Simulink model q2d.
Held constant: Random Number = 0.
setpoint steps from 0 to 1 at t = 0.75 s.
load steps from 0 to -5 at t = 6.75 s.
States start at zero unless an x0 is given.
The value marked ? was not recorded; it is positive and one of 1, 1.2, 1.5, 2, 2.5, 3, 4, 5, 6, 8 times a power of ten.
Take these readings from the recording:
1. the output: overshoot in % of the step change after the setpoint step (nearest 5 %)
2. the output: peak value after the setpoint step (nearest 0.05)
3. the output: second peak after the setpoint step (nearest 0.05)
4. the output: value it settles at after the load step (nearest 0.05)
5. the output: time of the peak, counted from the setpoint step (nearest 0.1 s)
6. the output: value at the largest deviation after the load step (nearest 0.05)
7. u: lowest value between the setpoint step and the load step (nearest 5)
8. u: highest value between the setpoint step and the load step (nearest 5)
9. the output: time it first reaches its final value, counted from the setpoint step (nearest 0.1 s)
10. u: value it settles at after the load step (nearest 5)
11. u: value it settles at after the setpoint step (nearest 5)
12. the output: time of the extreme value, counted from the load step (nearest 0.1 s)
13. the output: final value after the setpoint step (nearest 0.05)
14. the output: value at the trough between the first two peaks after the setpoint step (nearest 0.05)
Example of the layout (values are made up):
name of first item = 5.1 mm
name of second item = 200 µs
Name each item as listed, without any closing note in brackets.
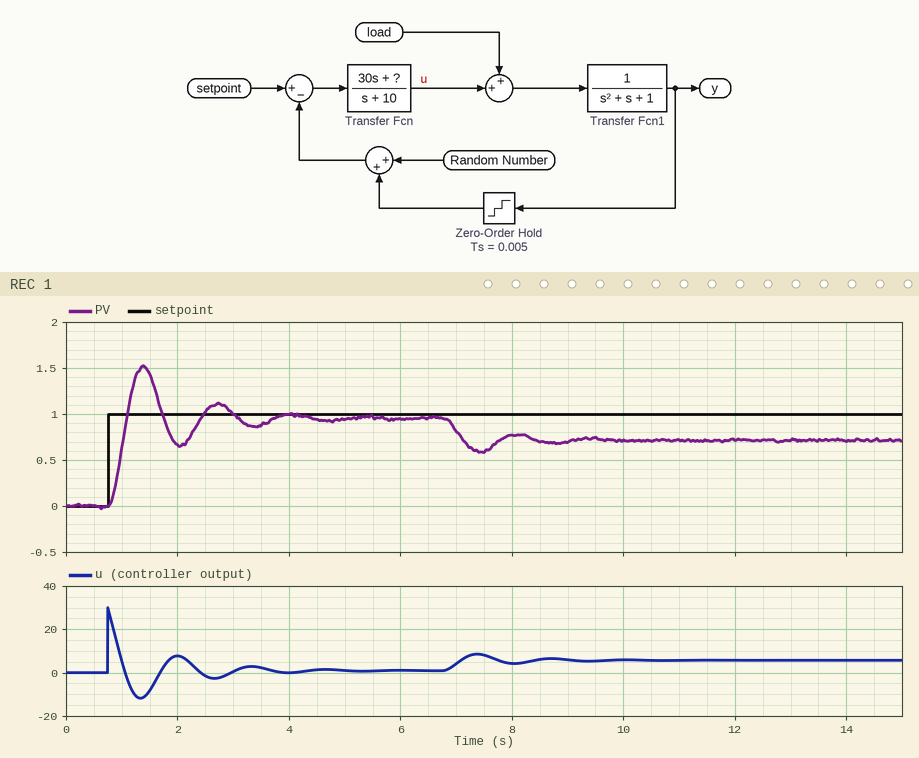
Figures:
the output: overshoot in % of the step change after the setpoint step = 60 %
the output: peak value after the setpoint step = 1.50
the output: second peak after the setpoint step = 1.10
the output: value it settles at after the load step = 0.70
the output: time of the peak, counted from the setpoint step = 0.6 s
the output: value at the largest deviation after the load step = 0.60
u: lowest value between the setpoint step and the load step = -10
u: highest value between the setpoint step and the load step = 30
the output: time it first reaches its final value, counted from the setpoint step = 0.3 s
u: value it settles at after the load step = 5
u: value it settles at after the setpoint step = 0
the output: time of the extreme value, counted from the load step = 0.7 s
the output: final value after the setpoint step = 0.95
the output: value at the trough between the first two peaks after the setpoint step = 0.65
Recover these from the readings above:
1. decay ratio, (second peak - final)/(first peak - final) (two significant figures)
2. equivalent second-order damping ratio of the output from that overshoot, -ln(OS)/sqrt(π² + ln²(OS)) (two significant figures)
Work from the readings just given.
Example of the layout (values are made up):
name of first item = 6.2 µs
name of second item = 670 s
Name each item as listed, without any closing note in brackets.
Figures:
decay ratio, (second peak - final)/(first peak - final) = 0.27
equivalent second-order damping ratio of the output from that overshoot, -ln(OS)/sqrt(π² + ln²(OS)) = 0.16
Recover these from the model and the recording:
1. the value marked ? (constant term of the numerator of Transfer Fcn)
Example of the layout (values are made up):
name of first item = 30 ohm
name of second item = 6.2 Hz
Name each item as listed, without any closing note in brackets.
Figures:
the value marked ? = 200
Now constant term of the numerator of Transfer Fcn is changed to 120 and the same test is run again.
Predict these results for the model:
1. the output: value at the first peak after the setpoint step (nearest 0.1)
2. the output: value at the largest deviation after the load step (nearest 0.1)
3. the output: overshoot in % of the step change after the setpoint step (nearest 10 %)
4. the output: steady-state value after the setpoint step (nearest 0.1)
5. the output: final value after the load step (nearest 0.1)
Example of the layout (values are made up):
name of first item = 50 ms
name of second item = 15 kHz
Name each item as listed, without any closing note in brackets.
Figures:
the output: value at the first peak after the setpoint step = 1.3
the output: value at the largest deviation after the load step = 0.4
the output: overshoot in % of the step change after the setpoint step = 40 %
the output: steady-state value after the setpoint step = 0.9
the output: final value after the load step = 0.5
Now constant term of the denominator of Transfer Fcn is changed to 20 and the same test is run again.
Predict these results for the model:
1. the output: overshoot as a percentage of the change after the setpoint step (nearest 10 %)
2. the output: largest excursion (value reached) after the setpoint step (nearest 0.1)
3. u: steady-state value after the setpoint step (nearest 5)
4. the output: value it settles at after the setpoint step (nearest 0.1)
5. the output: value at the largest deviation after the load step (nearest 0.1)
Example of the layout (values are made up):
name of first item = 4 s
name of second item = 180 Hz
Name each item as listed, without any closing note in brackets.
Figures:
the output: overshoot as a percentage of the change after the setpoint step = 40 %
the output: largest excursion (value reached) after the setpoint step = 1.3
u: steady-state value after the setpoint step = 0
the output: value it settles at after the setpoint step = 0.9
the output: value at the largest deviation after the load step = 0.3
